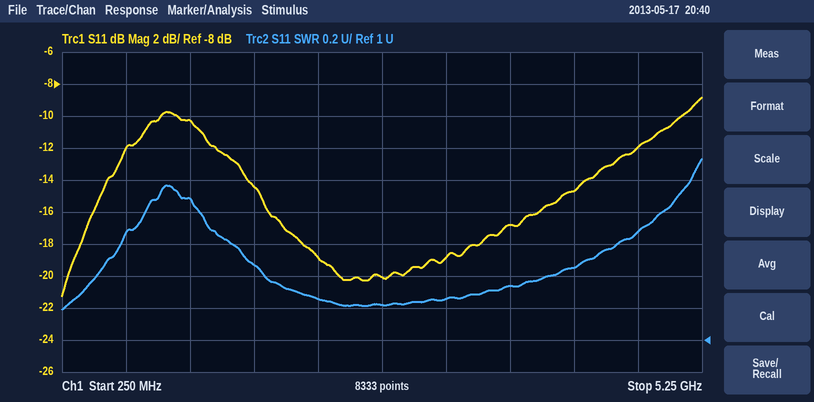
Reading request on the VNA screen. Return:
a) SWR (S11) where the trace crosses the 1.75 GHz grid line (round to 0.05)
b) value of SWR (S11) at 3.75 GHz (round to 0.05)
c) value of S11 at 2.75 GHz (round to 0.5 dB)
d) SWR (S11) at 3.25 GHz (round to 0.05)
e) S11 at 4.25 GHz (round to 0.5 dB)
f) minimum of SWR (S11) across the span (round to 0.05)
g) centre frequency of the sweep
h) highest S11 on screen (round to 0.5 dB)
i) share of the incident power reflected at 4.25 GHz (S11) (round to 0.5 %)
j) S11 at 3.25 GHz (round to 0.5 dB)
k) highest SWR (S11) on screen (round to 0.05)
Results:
1.45
1.35
-20.0 dB
1.25
-14.5 dB
1.20
2.75 GHz
-9.0 dB
3.5 %
-19.0 dB
2.15
